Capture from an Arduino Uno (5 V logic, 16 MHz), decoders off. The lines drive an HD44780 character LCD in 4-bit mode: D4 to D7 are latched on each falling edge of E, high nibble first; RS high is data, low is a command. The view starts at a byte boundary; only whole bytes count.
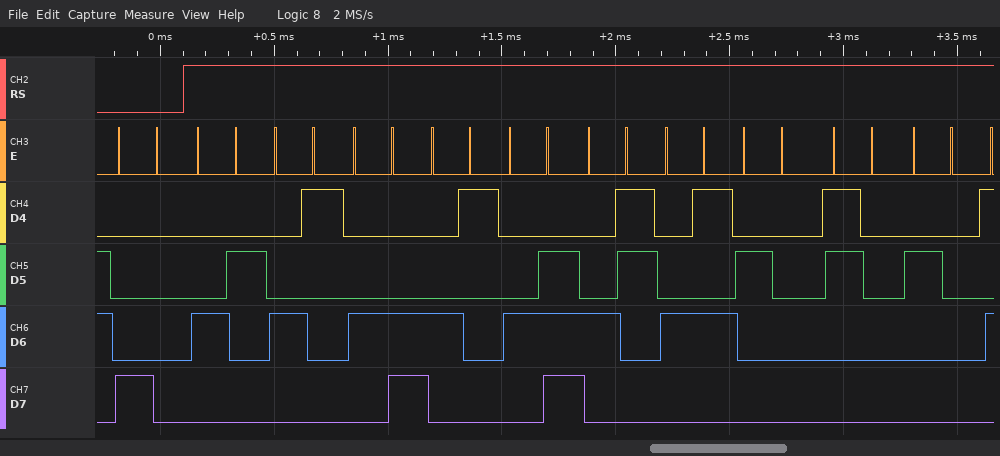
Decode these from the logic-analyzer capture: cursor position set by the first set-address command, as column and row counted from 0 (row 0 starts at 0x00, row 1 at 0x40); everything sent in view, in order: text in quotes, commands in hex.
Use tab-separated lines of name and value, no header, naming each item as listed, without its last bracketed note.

cursor position set by the first set-address command, as column and row counted from 0	column 0, row 0
everything sent in view, in order: text in quotes, commands in hex	0x80 "BALANCE 0 "
